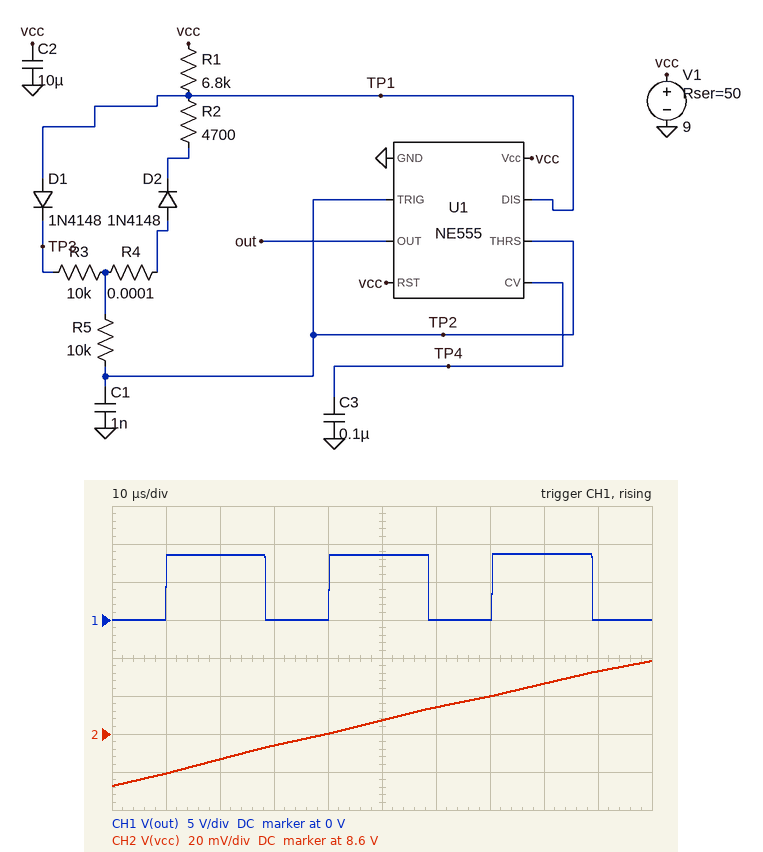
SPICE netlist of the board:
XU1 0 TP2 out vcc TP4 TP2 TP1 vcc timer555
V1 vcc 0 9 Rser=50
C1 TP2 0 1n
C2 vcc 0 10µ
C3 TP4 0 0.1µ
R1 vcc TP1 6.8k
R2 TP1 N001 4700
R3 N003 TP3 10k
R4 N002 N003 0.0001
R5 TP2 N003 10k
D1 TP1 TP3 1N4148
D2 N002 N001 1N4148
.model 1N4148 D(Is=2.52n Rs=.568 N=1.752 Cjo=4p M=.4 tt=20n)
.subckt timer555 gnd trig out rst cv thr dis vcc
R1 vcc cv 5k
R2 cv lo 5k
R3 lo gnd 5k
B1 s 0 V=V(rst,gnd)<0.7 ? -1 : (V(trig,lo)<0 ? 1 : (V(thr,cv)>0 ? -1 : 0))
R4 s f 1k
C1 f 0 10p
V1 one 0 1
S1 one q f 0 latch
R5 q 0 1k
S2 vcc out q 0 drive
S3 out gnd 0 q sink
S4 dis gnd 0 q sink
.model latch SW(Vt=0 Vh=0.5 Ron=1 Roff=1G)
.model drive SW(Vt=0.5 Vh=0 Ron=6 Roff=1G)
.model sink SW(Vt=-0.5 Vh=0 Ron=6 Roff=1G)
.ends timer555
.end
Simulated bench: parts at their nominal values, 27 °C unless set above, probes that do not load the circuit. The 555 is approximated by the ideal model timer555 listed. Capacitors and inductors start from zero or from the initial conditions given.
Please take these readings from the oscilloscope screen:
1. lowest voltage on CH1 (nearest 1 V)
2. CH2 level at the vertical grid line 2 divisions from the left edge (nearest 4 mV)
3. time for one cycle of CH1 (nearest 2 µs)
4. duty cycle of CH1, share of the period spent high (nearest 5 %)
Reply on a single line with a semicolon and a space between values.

0 V; 8.588 V; 30 µs; 60 %
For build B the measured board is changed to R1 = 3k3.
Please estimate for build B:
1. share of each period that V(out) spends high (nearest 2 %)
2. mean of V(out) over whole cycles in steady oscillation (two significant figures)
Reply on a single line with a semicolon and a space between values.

58 %; 5.0 V
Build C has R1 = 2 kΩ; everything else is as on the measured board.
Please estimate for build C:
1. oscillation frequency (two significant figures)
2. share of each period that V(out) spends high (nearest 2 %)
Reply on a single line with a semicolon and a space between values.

37 kHz; 56 %
